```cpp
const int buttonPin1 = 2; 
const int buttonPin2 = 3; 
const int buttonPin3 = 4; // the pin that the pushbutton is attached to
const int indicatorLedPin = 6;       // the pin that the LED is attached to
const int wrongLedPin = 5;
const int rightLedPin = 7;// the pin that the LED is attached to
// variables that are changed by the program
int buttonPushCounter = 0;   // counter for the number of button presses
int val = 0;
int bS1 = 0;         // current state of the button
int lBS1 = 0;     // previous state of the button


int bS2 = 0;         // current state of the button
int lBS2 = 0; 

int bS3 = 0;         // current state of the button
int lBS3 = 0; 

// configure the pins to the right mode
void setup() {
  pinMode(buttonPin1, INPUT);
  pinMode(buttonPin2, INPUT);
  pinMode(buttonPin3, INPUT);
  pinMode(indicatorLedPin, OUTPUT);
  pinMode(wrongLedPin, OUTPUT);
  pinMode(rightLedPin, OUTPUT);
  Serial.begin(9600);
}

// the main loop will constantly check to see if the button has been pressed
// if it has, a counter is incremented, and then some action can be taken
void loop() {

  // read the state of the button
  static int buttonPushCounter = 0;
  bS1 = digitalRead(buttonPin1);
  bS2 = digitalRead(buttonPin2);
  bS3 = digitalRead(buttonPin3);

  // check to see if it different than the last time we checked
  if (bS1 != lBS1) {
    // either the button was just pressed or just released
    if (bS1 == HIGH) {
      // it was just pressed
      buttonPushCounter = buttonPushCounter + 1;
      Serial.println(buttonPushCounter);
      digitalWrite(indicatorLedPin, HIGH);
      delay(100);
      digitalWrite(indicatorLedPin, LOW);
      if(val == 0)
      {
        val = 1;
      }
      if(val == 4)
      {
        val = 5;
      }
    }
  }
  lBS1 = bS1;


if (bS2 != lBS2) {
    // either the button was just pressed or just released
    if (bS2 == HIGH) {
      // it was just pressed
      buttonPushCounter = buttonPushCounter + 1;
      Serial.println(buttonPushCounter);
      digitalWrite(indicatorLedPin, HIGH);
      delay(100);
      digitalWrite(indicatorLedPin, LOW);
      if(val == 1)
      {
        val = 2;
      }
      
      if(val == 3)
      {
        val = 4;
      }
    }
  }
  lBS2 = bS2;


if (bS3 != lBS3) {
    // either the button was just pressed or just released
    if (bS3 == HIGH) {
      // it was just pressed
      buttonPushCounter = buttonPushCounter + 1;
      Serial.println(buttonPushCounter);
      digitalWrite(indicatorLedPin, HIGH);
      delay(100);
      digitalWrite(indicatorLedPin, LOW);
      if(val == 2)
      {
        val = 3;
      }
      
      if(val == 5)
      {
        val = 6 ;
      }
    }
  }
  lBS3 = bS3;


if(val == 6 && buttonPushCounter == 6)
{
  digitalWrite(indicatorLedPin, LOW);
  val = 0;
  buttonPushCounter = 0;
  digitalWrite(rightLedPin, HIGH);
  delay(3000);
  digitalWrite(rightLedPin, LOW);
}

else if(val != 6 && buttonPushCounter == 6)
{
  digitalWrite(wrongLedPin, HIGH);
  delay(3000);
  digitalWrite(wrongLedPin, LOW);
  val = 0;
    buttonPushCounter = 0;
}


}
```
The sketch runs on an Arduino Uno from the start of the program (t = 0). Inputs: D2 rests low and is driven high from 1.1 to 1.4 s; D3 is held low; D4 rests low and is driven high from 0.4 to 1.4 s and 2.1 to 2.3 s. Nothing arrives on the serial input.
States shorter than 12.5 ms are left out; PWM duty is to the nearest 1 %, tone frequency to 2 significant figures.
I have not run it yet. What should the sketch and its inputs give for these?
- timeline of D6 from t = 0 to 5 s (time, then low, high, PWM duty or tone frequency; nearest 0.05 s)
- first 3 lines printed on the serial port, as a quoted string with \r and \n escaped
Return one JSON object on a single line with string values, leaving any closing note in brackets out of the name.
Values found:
{"timeline of D6 from t = 0 to 5 s": "0 s low; 0.4 s high; 0.5 s low; 1.1 s high; 1.2 s low; 2.1 s high; 2.2 s low", "first 3 lines printed on the serial port, as a quoted string with \\r and \\n escaped": "\"1\\r\\n2\\r\\n3\\r\\n\""}
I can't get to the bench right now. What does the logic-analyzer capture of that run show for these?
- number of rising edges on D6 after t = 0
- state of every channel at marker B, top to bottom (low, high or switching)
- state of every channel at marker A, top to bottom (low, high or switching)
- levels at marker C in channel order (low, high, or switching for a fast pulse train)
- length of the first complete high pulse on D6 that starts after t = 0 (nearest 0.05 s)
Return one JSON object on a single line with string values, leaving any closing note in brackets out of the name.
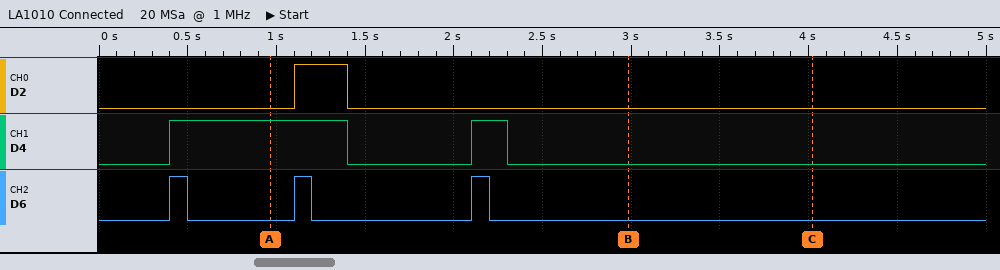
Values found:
{"number of rising edges on D6 after t = 0": "3", "state of every channel at marker B, top to bottom": "D2 low, D4 low, D6 low", "state of every channel at marker A, top to bottom": "D2 low, D4 high, D6 low", "levels at marker C in channel order": "D2 low, D4 low, D6 low", "length of the first complete high pulse on D6 that starts after t = 0": "0.10 s"}
